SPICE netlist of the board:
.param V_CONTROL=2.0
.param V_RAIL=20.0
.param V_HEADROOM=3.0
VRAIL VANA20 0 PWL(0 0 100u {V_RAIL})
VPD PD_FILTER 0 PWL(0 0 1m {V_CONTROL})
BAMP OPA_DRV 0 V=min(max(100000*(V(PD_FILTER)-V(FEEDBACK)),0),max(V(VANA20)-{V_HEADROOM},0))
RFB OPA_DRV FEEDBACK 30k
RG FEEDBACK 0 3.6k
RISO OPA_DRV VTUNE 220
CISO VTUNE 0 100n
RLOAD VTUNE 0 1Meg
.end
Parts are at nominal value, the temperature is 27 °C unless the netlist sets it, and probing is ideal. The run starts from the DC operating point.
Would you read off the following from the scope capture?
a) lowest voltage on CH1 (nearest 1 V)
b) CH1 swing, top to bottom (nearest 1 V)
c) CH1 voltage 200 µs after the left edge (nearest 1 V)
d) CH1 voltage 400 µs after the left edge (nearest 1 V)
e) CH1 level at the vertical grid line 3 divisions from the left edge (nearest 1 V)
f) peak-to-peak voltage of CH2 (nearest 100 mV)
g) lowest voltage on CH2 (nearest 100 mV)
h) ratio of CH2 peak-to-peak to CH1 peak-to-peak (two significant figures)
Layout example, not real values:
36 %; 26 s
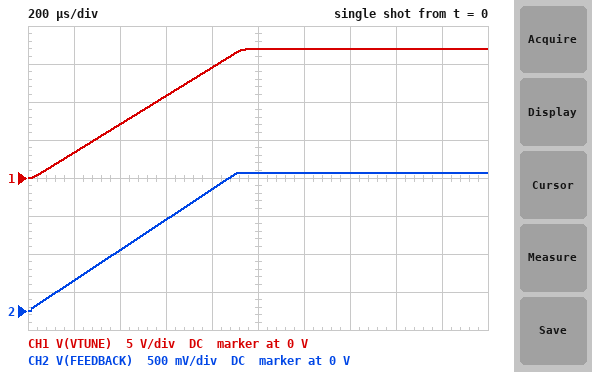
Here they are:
0 V; 17 V; 3 V; 7 V; 11 V; 1.8 V; 0 V; 0.11
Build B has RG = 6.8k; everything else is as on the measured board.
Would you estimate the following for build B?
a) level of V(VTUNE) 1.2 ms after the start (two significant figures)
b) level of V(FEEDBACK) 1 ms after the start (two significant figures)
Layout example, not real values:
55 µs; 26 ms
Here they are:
11 V; 2.0 V
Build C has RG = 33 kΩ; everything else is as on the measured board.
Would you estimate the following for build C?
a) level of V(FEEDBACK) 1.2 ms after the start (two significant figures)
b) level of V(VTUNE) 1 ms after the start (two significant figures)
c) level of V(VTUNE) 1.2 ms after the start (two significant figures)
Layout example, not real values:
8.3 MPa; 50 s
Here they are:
2.0 V; 3.7 V; 3.8 V
